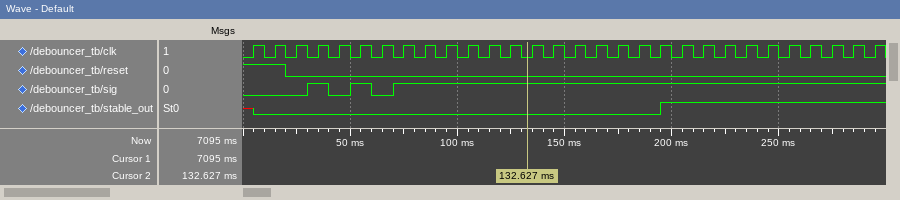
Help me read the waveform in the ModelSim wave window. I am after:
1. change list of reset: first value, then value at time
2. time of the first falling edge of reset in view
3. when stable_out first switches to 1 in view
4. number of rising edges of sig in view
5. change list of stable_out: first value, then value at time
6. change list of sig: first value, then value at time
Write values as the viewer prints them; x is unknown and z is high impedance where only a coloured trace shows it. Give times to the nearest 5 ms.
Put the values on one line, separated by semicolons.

1, 0 at 20 ms; 20 ms; 195 ms; 3; x, 0 at 5 ms, 1 at 195 ms; 0, 1 at 30 ms, 0 at 40 ms, 1 at 50 ms, 0 at 60 ms, 1 at 70 ms
